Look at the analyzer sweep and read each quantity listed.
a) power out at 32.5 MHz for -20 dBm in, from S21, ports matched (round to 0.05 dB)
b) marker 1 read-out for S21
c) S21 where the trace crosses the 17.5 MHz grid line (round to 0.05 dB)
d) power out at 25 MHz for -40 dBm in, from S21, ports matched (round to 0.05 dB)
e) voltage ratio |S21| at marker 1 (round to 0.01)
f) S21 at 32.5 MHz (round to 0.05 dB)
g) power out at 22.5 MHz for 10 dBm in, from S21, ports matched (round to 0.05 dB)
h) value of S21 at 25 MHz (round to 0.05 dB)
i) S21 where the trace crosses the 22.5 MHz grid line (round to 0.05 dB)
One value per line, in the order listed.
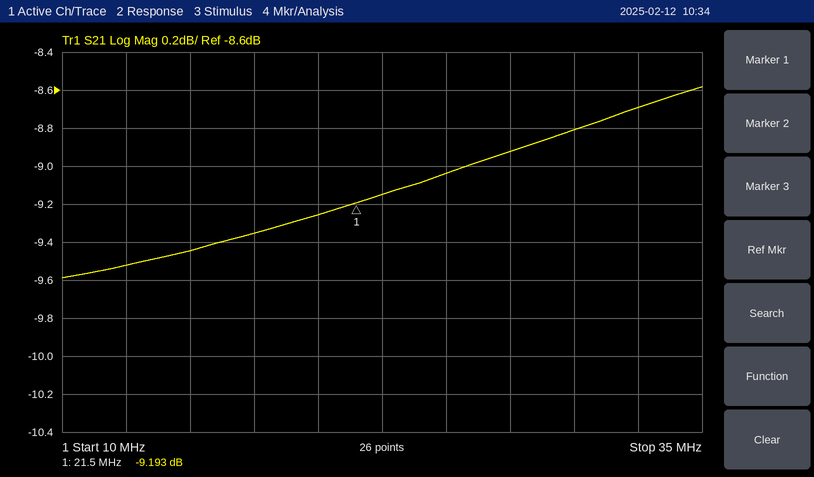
-28.70 dBm
-9.193 dB
-9.35 dB
-49.05 dBm
0.35
-8.70 dB
0.85 dBm
-9.05 dB
-9.15 dB
